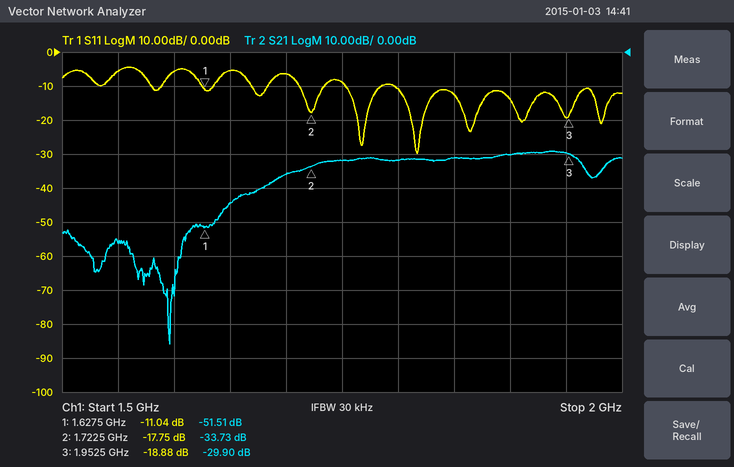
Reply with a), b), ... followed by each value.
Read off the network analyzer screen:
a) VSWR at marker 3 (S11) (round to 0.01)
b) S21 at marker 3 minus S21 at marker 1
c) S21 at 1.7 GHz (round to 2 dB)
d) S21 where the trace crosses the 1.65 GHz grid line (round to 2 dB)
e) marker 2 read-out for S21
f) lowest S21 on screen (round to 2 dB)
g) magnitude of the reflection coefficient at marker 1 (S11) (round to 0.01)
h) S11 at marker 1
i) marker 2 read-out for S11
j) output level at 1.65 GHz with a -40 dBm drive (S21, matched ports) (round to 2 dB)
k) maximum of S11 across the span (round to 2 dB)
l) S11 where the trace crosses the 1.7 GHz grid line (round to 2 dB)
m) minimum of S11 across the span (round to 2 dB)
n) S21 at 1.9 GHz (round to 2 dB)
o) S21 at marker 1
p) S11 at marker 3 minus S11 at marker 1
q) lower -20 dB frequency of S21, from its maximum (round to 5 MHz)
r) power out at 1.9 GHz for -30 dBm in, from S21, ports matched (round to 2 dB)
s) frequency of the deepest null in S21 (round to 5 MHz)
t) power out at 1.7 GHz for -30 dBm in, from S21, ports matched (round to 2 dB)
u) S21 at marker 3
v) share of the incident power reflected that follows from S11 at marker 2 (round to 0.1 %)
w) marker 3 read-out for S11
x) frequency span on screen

a) 1.26
b) 21.61 dB
c) -36 dB
d) -44 dB
e) -33.73 dB
f) -86 dB
g) 0.28
h) -11.04 dB
i) -17.75 dB
j) -84 dBm
k) -4 dB
l) -6 dB
m) -30 dB
n) -30 dB
o) -51.51 dB
p) -7.84 dB
q) 1.640 GHz
r) -60 dBm
s) 1.595 GHz
t) -66 dBm
u) -29.90 dB
v) 1.7 %
w) -18.88 dB
x) 500 MHz
